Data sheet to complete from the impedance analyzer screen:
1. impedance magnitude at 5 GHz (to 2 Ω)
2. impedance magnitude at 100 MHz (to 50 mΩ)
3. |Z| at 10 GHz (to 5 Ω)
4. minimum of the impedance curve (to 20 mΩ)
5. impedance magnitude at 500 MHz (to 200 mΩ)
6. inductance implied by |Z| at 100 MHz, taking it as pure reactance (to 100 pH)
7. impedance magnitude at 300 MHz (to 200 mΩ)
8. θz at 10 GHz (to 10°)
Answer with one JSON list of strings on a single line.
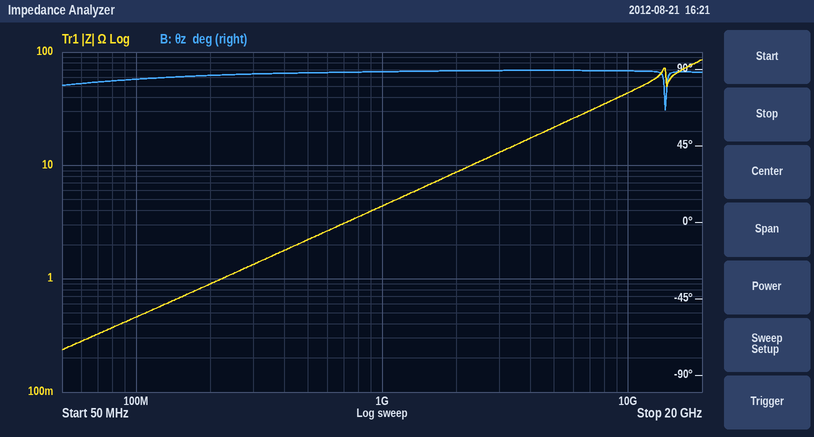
["22 Ω", "450 mΩ", "45 Ω", "240 mΩ", "2.2 Ω", "700 pH", "1.4 Ω", "90°"]
